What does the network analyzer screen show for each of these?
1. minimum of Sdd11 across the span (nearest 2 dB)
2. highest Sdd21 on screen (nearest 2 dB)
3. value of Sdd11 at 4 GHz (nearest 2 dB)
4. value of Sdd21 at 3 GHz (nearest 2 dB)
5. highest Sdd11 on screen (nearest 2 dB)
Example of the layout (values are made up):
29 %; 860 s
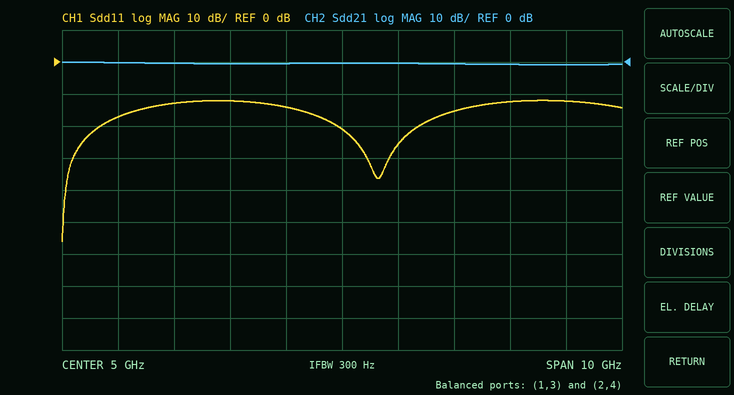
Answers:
-56 dB; 0 dB; -14 dB; 0 dB; -12 dB
